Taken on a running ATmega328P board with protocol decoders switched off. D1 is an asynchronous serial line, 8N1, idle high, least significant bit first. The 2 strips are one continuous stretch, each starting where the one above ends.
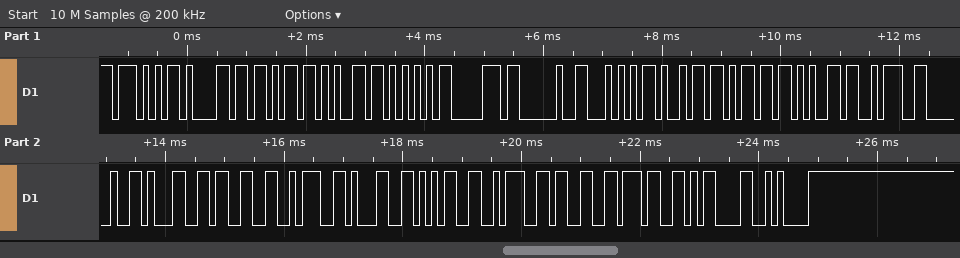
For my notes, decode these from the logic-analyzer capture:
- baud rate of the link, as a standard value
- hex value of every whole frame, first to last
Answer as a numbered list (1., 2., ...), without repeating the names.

1. 9600 baud
2. 57 61 6B 65 55 70 20 54 69 6D 65 3A 20 31 33 3A 31 35 3A 33 37 0D 0A
